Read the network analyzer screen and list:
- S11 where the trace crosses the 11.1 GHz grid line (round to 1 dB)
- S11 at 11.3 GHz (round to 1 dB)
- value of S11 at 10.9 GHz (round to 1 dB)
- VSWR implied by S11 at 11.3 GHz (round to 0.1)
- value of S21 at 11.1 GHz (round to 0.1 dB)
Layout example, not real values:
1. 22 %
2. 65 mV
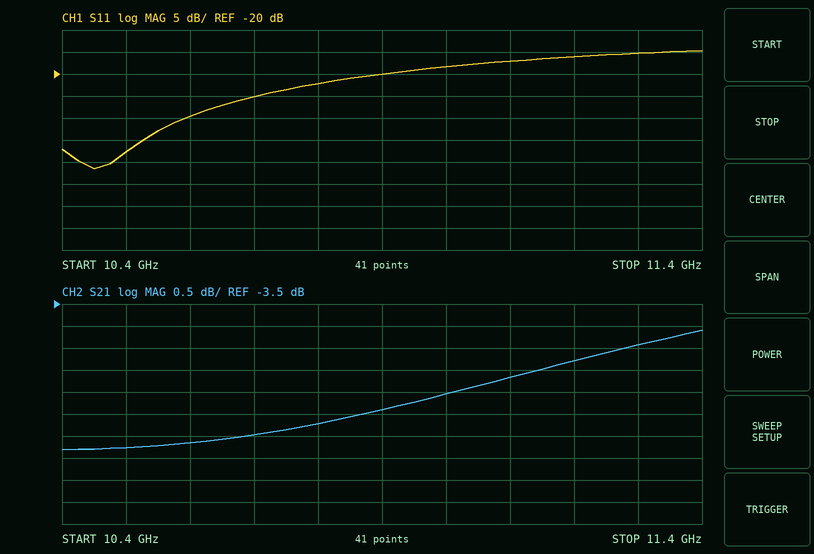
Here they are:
1. -17 dB
2. -15 dB
3. -20 dB
4. 1.4
5. -5.2 dB
